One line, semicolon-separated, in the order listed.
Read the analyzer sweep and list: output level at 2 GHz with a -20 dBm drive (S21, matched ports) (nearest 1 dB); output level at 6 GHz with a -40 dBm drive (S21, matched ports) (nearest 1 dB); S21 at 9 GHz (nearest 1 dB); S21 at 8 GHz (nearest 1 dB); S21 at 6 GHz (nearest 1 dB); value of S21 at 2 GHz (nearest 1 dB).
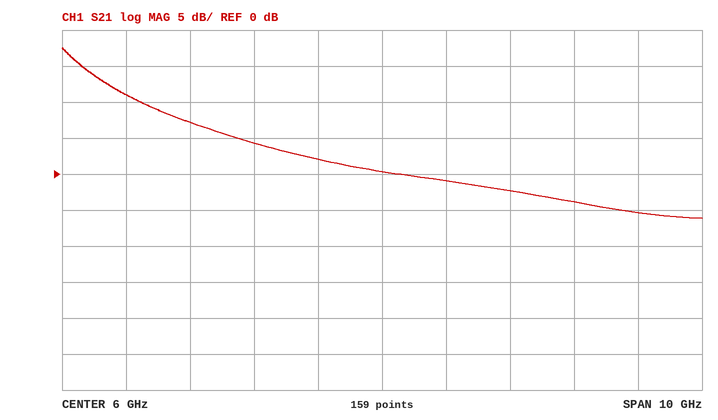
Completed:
-9 dBm; -40 dBm; -4 dB; -2 dB; 0 dB; 11 dB
